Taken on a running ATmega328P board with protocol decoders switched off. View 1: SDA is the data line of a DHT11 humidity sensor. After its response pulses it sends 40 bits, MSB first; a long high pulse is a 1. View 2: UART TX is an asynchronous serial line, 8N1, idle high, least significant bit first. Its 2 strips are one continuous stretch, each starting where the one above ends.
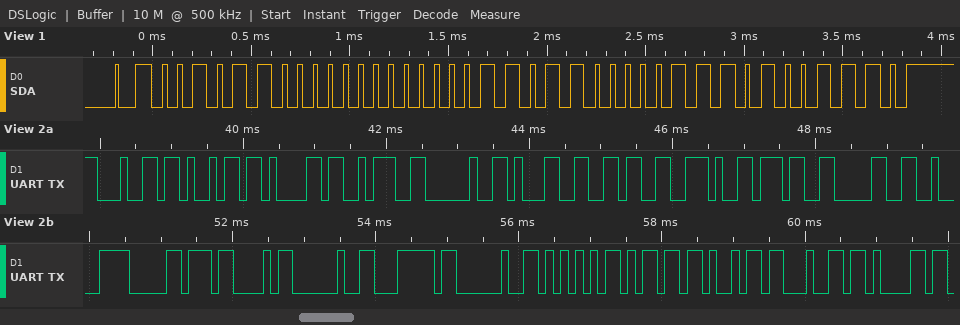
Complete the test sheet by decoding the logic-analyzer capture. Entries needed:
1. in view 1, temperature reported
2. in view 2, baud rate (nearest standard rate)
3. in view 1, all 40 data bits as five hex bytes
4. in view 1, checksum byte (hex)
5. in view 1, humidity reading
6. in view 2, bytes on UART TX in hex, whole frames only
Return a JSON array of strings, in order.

["27.7 °C", "9600 baud", "2C 00 1B 07 4E", "0x4E", "44 %", "64 69 61 3A 20 31 36 2E 37 30 C2 B0 43 20 7C 20 55 6D 69 64 61"]
